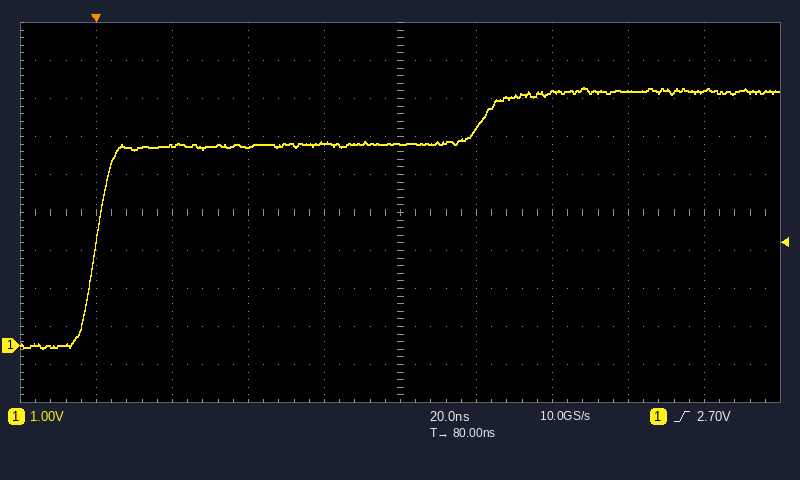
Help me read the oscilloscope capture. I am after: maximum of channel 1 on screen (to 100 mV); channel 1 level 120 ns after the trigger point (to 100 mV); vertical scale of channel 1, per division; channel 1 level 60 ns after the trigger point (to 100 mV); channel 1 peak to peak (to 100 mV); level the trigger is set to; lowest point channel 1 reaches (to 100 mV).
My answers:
6.8 V
6.7 V
1 V
5.3 V
6.9 V
2.70 V
-100 mV
